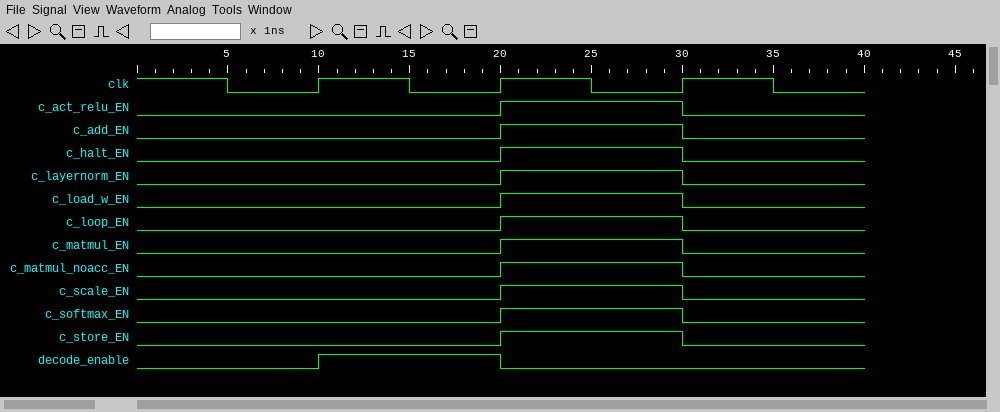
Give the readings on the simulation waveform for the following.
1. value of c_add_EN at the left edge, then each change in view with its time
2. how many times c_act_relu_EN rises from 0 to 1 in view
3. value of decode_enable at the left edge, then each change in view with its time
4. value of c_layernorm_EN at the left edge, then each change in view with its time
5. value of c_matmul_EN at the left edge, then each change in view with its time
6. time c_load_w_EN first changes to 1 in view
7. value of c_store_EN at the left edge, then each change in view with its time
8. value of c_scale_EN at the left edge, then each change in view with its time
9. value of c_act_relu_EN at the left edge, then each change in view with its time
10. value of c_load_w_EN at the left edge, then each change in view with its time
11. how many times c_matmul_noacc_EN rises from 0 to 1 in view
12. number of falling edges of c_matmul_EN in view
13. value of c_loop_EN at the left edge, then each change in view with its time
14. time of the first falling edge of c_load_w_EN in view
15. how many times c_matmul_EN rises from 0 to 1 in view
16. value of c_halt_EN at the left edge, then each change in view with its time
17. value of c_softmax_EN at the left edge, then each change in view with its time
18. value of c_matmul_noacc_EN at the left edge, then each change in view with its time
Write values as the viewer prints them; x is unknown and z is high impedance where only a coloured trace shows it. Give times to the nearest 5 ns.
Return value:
0, 1 at 20 ns, 0 at 30 ns
1
0, 1 at 10 ns, 0 at 20 ns
0, 1 at 20 ns, 0 at 30 ns
0, 1 at 20 ns, 0 at 30 ns
20 ns
0, 1 at 20 ns, 0 at 30 ns
0, 1 at 20 ns, 0 at 30 ns
0, 1 at 20 ns, 0 at 30 ns
0, 1 at 20 ns, 0 at 30 ns
1
1
0, 1 at 20 ns, 0 at 30 ns
30 ns
1
0, 1 at 20 ns, 0 at 30 ns
0, 1 at 20 ns, 0 at 30 ns
0, 1 at 20 ns, 0 at 30 ns
